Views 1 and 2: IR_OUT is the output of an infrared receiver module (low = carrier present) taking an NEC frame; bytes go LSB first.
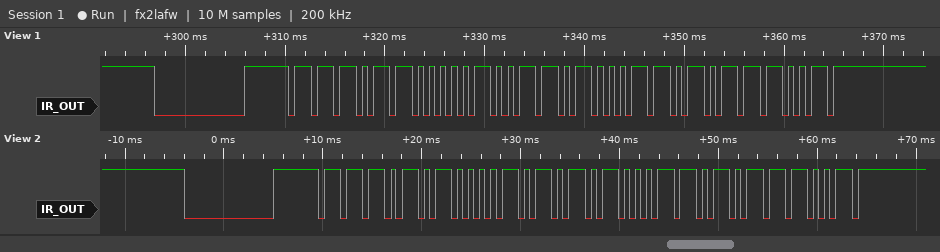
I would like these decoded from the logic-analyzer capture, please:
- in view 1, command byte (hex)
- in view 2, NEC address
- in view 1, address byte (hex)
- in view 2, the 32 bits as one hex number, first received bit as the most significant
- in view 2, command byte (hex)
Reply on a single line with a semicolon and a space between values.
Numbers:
0x62; 0x57; 0x37; 0xEA1546B9; 0x62
